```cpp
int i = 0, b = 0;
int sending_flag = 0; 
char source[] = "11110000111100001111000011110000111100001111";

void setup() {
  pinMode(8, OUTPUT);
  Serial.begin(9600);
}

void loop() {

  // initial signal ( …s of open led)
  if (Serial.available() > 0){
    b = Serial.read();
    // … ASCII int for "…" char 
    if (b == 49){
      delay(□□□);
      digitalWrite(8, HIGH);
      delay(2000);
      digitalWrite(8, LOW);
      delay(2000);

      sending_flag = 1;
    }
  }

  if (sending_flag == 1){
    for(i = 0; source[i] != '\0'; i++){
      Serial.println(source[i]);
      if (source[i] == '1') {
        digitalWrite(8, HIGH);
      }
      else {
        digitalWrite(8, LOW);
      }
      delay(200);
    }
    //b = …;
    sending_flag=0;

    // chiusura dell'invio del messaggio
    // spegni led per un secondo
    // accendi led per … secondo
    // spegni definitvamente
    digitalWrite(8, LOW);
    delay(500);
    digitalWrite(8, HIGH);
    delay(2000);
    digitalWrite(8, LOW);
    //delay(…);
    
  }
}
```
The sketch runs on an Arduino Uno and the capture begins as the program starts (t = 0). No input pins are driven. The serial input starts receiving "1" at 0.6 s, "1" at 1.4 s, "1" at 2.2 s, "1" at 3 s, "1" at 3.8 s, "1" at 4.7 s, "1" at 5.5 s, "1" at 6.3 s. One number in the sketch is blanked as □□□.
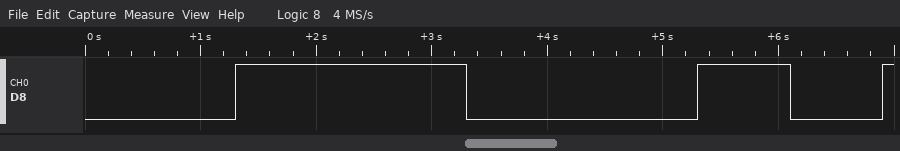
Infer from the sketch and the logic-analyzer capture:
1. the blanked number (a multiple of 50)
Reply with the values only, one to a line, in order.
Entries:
700
